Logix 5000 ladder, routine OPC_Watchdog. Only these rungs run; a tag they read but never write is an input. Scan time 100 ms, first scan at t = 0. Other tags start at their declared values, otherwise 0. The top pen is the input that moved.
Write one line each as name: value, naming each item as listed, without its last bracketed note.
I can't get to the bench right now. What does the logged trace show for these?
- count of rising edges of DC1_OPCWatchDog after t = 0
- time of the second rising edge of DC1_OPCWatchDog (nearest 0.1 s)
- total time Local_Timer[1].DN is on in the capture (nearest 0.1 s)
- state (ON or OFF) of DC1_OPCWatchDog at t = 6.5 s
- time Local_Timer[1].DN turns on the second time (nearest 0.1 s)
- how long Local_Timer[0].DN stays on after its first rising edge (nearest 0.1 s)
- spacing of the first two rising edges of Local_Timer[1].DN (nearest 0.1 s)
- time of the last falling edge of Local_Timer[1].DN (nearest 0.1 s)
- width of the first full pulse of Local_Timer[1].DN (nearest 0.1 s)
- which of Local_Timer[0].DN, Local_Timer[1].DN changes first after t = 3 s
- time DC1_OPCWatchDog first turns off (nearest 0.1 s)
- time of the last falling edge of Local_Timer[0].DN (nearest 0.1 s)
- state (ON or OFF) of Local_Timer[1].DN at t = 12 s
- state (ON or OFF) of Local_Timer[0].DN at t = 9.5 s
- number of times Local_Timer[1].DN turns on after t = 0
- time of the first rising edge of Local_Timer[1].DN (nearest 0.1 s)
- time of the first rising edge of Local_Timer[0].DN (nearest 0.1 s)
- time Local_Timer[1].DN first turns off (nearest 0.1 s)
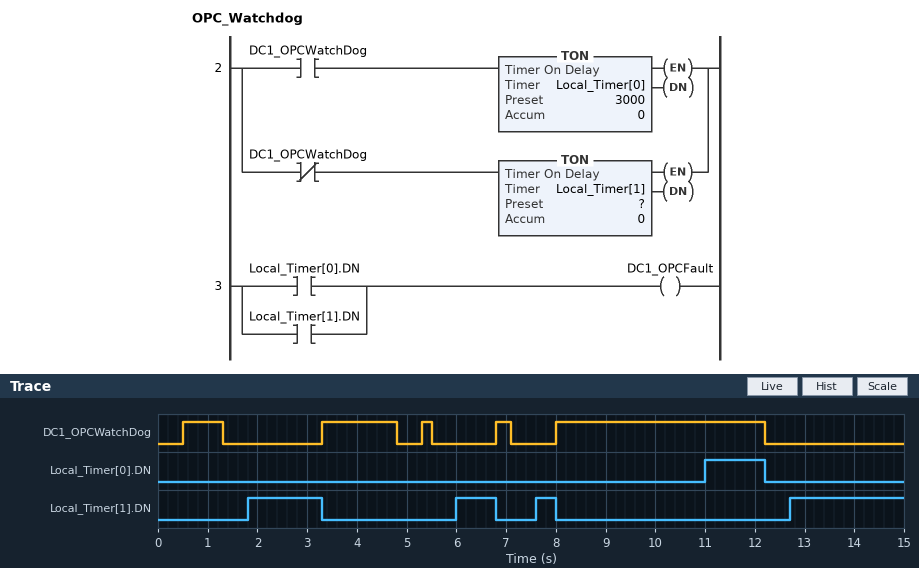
count of rising edges of DC1_OPCWatchDog after t = 0: 5
time of the second rising edge of DC1_OPCWatchDog: 3.3 s
total time Local_Timer[1].DN is on in the capture: 5.0 s
state (ON or OFF) of DC1_OPCWatchDog at t = 6.5 s: OFF
time Local_Timer[1].DN turns on the second time: 6.0 s
how long Local_Timer[0].DN stays on after its first rising edge: 1.2 s
spacing of the first two rising edges of Local_Timer[1].DN: 4.2 s
time of the last falling edge of Local_Timer[1].DN: 8.0 s
width of the first full pulse of Local_Timer[1].DN: 1.5 s
which of Local_Timer[0].DN, Local_Timer[1].DN changes first after t = 3 s: Local_Timer[1].DN
time DC1_OPCWatchDog first turns off: 1.3 s
time of the last falling edge of Local_Timer[0].DN: 12.2 s
state (ON or OFF) of Local_Timer[1].DN at t = 12 s: OFF
state (ON or OFF) of Local_Timer[0].DN at t = 9.5 s: OFF
number of times Local_Timer[1].DN turns on after t = 0: 4
time of the first rising edge of Local_Timer[1].DN: 1.8 s
time of the first rising edge of Local_Timer[0].DN: 11.0 s
time Local_Timer[1].DN first turns off: 3.3 s
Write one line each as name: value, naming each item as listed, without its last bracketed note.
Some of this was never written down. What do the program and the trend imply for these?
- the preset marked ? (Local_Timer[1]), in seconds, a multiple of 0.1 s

the preset marked ? (Local_Timer[1]), in seconds, a multiple of 0.1 s: 0.5 s
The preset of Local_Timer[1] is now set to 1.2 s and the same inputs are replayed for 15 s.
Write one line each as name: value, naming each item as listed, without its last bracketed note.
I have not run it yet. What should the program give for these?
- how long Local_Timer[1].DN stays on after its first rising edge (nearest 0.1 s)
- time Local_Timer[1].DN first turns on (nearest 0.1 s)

how long Local_Timer[1].DN stays on after its first rising edge: 0.8 s
time Local_Timer[1].DN first turns on: 2.5 s
